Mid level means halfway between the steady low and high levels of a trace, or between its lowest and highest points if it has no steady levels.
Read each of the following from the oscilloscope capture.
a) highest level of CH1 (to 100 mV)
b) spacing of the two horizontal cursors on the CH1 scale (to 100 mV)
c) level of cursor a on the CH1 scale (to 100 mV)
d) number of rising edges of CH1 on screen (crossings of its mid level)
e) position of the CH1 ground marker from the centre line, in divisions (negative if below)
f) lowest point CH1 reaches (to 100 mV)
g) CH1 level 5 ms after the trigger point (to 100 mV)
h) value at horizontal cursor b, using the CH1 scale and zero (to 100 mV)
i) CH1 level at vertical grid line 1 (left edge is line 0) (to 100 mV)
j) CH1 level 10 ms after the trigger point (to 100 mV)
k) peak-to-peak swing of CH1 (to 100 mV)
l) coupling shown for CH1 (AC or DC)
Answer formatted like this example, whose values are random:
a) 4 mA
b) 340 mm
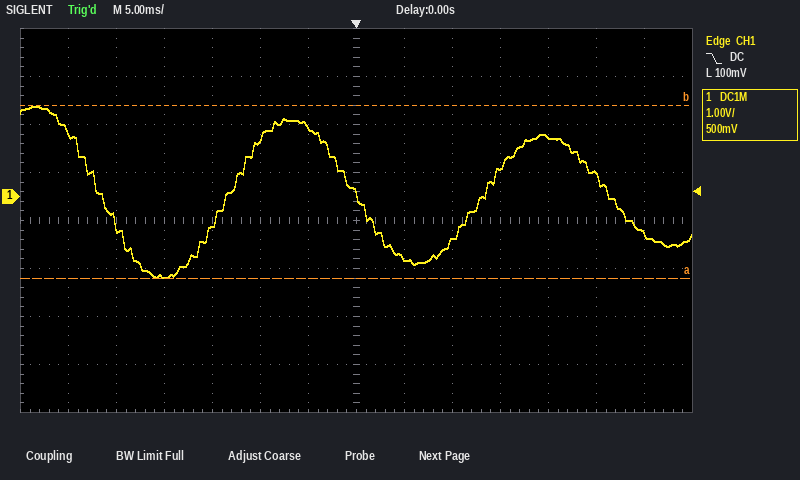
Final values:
a) 1.9 V
b) 3.6 V
c) -1.7 V
d) 2
e) +0.5 div
f) -1.7 V
g) -1.3 V
h) 1.9 V
i) 1.3 V
j) -900 mV
k) 3.6 V
l) DC
